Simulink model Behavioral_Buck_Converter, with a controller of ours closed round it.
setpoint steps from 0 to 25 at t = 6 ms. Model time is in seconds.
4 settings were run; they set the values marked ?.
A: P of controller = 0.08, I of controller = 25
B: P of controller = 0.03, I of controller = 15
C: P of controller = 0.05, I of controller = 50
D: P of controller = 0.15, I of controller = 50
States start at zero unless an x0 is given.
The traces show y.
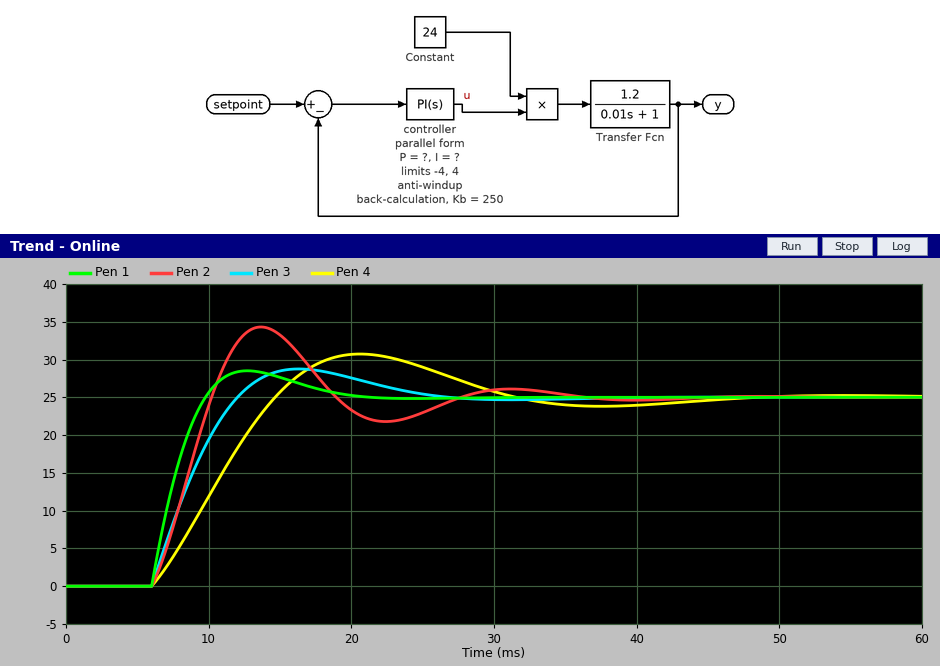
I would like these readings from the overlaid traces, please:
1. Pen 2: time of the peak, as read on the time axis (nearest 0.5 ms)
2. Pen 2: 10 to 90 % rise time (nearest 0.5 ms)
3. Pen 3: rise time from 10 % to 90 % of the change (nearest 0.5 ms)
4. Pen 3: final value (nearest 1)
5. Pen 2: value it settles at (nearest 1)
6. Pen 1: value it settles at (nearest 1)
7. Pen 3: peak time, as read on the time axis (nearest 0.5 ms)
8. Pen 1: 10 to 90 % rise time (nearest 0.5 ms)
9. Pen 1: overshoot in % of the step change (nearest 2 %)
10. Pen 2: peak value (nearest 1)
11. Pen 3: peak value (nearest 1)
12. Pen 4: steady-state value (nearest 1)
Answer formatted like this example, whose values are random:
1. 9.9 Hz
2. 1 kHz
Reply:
1. 13.5 ms
2. 3.0 ms
3. 4.5 ms
4. 25
5. 25
6. 25
7. 16.5 ms
8. 3.0 ms
9. 14 %
10. 34
11. 29
12. 25
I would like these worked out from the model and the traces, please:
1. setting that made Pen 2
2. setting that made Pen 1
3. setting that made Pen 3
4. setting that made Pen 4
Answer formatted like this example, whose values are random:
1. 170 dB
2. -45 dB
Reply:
1. C
2. D
3. A
4. B
